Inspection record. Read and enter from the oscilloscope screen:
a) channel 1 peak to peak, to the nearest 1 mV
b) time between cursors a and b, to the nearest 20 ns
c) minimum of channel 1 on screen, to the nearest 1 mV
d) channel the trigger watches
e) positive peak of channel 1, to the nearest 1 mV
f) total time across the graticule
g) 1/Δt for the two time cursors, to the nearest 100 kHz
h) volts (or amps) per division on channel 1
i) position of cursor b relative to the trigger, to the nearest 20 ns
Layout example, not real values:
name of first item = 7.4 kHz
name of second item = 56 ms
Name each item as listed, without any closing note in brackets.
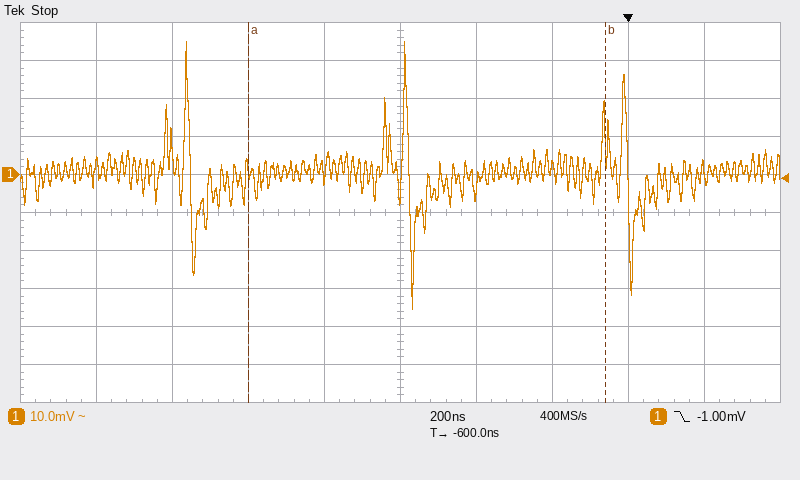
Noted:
channel 1 peak to peak, to the nearest 1 mV = 70 mV
time between cursors a and b, to the nearest 20 ns = 940 ns
minimum of channel 1 on screen, to the nearest 1 mV = -35 mV
channel the trigger watches = channel 1
positive peak of channel 1, to the nearest 1 mV = 35 mV
total time across the graticule = 2 µs
1/Δt for the two time cursors, to the nearest 100 kHz = 1.1 MHz
volts (or amps) per division on channel 1 = 10 mV
position of cursor b relative to the trigger, to the nearest 20 ns = -60 ns
